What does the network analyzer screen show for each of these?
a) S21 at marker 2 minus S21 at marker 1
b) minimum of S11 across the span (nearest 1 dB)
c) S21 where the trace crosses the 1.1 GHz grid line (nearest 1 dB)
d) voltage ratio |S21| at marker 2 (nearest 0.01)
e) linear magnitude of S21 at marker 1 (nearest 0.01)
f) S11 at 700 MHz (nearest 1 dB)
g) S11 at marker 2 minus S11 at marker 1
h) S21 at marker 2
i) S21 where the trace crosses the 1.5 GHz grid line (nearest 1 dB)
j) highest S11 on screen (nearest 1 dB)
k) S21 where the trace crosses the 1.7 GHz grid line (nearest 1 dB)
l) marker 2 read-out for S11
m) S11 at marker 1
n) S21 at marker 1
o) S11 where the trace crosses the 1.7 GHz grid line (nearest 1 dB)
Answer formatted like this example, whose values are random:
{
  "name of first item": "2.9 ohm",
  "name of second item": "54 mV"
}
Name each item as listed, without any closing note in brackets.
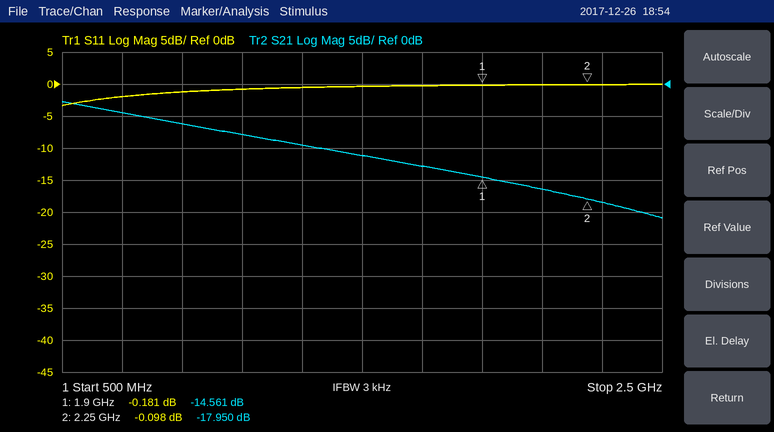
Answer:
{
  "S21 at marker 2 minus S21 at marker 1": "-3.389 dB",
  "minimum of S11 across the span": "-3 dB",
  "S21 where the trace crosses the 1.1 GHz grid line": "-8 dB",
  "voltage ratio |S21| at marker 2": "0.13",
  "linear magnitude of S21 at marker 1": "0.19",
  "S11 at 700 MHz": "-2 dB",
  "S11 at marker 2 minus S11 at marker 1": "0.083 dB",
  "S21 at marker 2": "-17.950 dB",
  "S21 where the trace crosses the 1.5 GHz grid line": "-11 dB",
  "highest S11 on screen": "0 dB",
  "S21 where the trace crosses the 1.7 GHz grid line": "-13 dB",
  "marker 2 read-out for S11": "-0.098 dB",
  "S11 at marker 1": "-0.181 dB",
  "S21 at marker 1": "-14.561 dB",
  "S11 where the trace crosses the 1.7 GHz grid line": "0 dB"
}
